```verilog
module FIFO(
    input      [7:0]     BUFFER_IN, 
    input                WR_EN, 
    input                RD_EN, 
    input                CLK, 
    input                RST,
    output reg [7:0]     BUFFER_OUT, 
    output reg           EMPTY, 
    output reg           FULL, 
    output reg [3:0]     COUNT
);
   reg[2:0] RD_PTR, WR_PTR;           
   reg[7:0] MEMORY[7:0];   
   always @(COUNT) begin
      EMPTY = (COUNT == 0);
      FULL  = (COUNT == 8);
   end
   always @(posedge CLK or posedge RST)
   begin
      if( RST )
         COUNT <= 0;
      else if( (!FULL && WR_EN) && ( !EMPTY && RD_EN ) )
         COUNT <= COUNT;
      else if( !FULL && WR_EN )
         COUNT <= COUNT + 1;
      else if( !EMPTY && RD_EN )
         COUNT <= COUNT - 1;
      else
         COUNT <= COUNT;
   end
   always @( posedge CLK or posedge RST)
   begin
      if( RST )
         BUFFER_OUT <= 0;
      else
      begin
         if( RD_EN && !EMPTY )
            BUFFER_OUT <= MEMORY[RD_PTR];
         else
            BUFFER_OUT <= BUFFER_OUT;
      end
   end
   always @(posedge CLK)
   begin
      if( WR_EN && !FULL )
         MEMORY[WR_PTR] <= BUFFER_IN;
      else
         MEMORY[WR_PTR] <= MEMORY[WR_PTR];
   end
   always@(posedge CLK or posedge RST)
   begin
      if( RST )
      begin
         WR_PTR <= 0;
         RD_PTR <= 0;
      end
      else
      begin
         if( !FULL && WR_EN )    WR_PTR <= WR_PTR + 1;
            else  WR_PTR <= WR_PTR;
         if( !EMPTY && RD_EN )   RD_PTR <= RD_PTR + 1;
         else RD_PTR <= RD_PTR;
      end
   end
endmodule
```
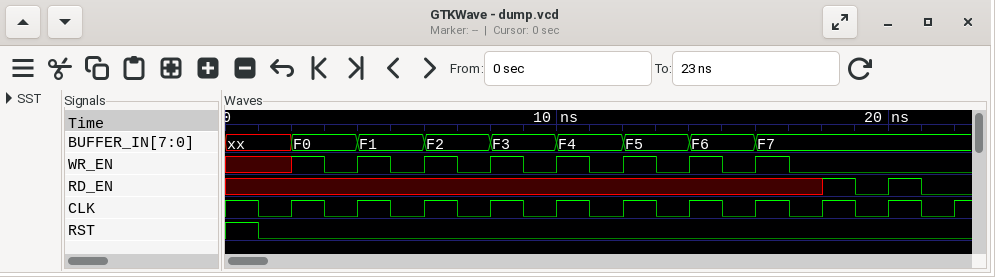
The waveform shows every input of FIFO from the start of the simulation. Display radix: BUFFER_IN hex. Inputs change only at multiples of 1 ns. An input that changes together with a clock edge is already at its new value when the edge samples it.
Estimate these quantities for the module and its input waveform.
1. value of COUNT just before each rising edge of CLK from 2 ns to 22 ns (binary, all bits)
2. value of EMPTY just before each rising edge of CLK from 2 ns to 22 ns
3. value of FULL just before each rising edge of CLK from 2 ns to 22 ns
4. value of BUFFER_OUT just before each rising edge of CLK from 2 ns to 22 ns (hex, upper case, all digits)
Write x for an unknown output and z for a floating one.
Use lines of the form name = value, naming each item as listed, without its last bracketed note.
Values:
value of COUNT just before each rising edge of CLK from 2 ns to 22 ns = 0000, 0001, 0010, 0011, 0100, 0101, 0110, 0111, 1000, 0111, 0110
value of EMPTY just before each rising edge of CLK from 2 ns to 22 ns = 1 0 0 0 0 0 0 0 0 0 0
value of FULL just before each rising edge of CLK from 2 ns to 22 ns = 0 0 0 0 0 0 0 0 1 0 0
value of BUFFER_OUT just before each rising edge of CLK from 2 ns to 22 ns = 00, 00, 00, 00, 00, 00, 00, 00, 00, F0, F1
